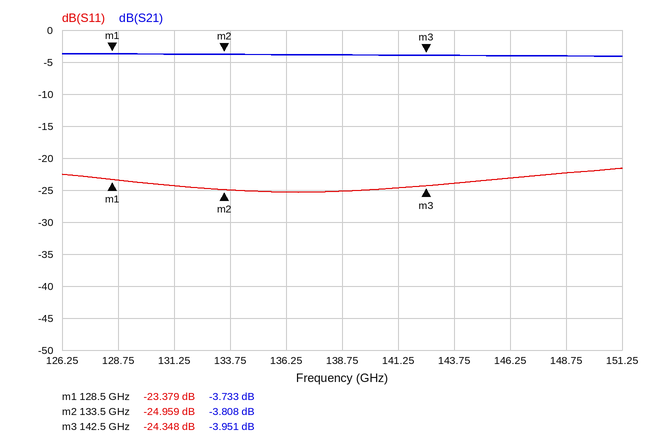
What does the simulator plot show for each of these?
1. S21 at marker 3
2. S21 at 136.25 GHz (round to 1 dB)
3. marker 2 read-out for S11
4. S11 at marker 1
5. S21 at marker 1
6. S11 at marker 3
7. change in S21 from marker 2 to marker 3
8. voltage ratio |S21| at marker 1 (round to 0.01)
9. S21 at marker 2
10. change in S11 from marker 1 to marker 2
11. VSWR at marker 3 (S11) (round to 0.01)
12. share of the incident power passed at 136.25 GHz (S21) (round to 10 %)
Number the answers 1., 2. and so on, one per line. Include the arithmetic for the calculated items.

1. -3.951 dB
2. -4 dB
3. -24.959 dB
4. -23.379 dB
5. -3.733 dB
6. -24.348 dB
7. -3.951 − (-3.808) = -0.143 dB
8. 10^(-3.733/20) ≈ 0.65
9. -3.808 dB
10. -24.959 − (-23.379) = -1.580 dB
11. (1 + 0.0606)/(1 − 0.0606) ≈ 1.13
12. 10^(-4/10) ≈ 40 %
